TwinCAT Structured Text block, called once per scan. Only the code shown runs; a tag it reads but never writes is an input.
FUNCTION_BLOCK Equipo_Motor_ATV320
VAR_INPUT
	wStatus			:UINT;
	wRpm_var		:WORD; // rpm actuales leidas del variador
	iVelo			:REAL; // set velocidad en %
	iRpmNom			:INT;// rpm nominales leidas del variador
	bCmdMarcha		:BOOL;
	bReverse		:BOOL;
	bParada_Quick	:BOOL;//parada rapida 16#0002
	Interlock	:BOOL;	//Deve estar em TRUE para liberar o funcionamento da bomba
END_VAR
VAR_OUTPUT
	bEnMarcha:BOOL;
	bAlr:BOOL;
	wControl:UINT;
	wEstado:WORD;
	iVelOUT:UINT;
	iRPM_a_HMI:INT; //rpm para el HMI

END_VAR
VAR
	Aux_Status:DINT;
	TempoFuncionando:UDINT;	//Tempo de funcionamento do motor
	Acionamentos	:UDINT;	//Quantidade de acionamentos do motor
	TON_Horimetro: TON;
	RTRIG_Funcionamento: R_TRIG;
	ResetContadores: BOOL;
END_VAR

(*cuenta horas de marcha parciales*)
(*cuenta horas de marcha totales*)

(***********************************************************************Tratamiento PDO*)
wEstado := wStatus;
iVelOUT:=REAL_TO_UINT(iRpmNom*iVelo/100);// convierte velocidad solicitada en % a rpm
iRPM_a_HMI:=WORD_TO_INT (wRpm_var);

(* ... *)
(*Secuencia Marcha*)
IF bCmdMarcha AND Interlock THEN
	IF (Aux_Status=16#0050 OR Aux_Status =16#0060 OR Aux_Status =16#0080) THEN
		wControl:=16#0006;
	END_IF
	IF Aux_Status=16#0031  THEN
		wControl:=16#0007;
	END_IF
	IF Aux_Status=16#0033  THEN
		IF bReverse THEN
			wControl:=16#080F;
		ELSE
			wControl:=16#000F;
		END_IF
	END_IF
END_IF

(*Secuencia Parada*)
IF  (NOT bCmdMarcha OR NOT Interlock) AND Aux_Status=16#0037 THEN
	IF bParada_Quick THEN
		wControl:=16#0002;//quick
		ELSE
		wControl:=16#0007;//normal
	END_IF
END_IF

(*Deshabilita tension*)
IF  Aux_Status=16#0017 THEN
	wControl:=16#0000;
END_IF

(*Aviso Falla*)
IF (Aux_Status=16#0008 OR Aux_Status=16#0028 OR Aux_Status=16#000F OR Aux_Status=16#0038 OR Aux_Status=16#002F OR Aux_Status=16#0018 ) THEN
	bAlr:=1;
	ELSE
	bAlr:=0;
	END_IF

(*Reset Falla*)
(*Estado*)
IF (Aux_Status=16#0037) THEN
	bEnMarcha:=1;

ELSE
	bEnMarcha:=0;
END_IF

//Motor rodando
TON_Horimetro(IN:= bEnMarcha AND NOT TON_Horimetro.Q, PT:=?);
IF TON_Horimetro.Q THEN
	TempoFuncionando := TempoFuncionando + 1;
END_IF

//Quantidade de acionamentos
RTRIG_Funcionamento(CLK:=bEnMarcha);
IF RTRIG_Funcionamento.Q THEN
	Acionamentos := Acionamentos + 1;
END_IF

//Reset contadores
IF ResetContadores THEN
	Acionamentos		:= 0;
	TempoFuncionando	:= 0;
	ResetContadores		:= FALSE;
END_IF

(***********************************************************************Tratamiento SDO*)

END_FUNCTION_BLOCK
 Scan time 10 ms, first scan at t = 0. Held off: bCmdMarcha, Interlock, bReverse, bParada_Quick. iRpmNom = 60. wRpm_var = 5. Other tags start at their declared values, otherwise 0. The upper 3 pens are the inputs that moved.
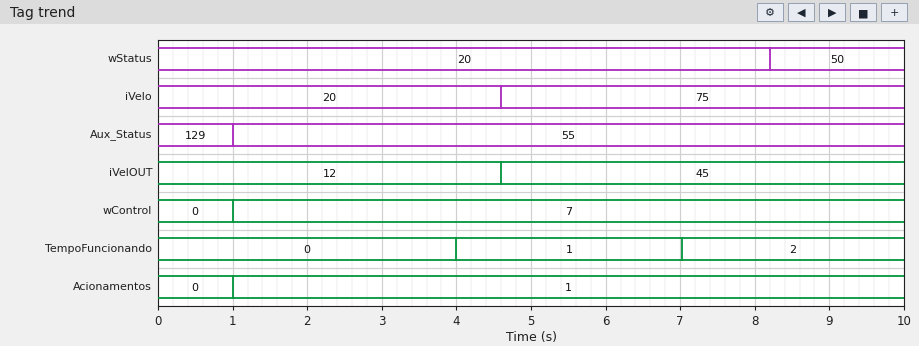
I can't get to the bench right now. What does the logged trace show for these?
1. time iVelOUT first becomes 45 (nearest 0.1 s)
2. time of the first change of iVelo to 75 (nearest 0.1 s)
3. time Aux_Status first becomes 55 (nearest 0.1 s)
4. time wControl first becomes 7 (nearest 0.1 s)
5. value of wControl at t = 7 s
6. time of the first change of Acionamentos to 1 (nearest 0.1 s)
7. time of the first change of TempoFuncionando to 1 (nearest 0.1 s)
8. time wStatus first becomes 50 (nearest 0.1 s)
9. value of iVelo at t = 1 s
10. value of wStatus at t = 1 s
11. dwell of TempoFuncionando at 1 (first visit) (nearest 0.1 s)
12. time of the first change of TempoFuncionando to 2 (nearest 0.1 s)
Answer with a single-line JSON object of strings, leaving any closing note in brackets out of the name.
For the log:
{"time iVelOUT first becomes 45": "4.6 s", "time of the first change of iVelo to 75": "4.6 s", "time Aux_Status first becomes 55": "1.0 s", "time wControl first becomes 7": "1.0 s", "value of wControl at t = 7 s": "7", "time of the first change of Acionamentos to 1": "1.0 s", "time of the first change of TempoFuncionando to 1": "4.0 s", "time wStatus first becomes 50": "8.2 s", "value of iVelo at t = 1 s": "20", "value of wStatus at t = 1 s": "20", "dwell of TempoFuncionando at 1 (first visit)": "3.0 s", "time of the first change of TempoFuncionando to 2": "7.0 s"}
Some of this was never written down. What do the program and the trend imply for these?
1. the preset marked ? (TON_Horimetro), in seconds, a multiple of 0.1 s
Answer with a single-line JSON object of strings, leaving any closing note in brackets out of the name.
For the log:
{"the preset marked ? (TON_Horimetro), in seconds, a multiple of 0.1 s": "3.0 s"}
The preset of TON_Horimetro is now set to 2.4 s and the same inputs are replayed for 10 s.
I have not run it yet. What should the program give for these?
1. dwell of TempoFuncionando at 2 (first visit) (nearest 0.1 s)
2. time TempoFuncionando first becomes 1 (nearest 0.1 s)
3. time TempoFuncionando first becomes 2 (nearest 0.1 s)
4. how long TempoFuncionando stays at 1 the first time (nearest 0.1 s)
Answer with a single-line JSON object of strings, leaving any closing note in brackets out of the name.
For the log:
{"dwell of TempoFuncionando at 2 (first visit)": "2.4 s", "time TempoFuncionando first becomes 1": "3.4 s", "time TempoFuncionando first becomes 2": "5.8 s", "how long TempoFuncionando stays at 1 the first time": "2.4 s"}
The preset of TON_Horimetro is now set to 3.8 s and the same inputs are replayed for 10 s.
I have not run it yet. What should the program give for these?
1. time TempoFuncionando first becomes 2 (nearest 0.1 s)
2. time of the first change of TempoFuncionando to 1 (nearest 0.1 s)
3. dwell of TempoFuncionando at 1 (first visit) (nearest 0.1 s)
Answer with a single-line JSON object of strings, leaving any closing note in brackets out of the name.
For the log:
{"time TempoFuncionando first becomes 2": "8.6 s", "time of the first change of TempoFuncionando to 1": "4.8 s", "dwell of TempoFuncionando at 1 (first visit)": "3.8 s"}
